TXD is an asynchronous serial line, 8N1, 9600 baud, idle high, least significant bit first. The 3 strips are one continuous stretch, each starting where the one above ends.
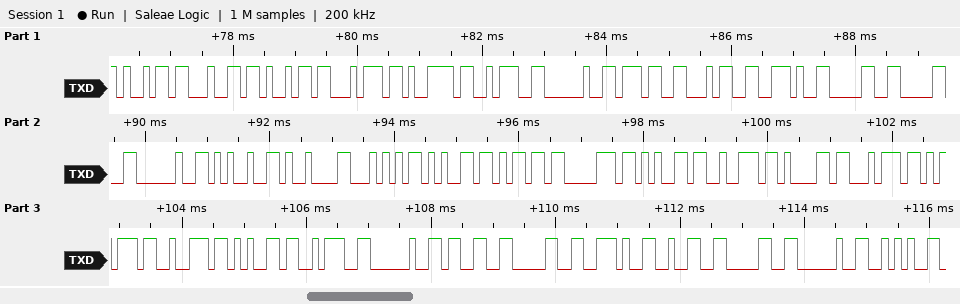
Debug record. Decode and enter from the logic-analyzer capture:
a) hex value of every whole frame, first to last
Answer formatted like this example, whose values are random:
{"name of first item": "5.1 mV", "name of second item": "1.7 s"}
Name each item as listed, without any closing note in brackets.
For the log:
{"hex value of every whole frame, first to last": "69 64 69 74 79 3A 20 37 34 2E 30 30 20 25 09 54 65 6D 70 65 72 61 74 75 72 65 3A 20 33 30 2E 32 30 20 2A"}
